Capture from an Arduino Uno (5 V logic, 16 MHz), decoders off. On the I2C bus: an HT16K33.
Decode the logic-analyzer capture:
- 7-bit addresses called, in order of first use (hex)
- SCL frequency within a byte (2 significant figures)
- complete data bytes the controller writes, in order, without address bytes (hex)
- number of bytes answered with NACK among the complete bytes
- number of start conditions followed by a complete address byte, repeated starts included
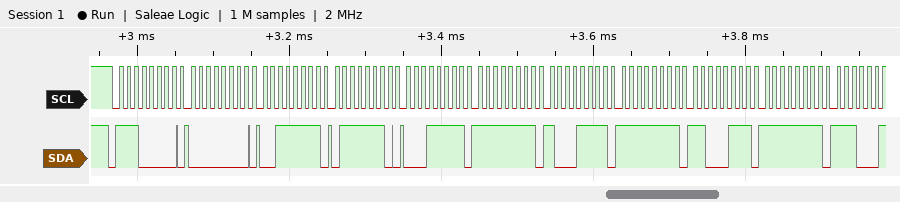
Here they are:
0x70
100 kHz
00 3F 7E 1F FF 8F FF C7 FF
0
1
